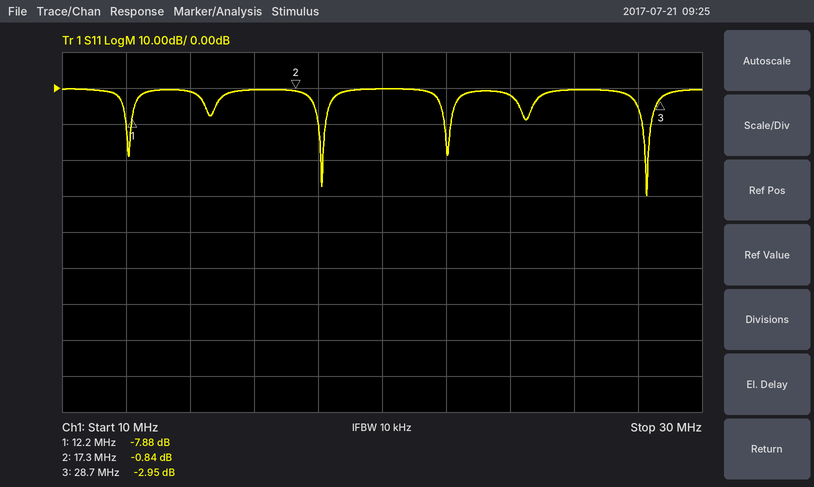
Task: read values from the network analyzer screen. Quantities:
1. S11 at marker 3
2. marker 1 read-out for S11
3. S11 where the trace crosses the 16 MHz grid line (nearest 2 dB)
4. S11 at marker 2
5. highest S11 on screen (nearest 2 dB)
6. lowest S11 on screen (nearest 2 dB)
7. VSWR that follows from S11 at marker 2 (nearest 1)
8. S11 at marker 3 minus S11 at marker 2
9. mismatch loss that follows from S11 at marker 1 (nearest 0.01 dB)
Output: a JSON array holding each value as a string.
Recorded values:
["-2.95 dB", "-7.88 dB", "0 dB", "-0.84 dB", "0 dB", "-30 dB", "21", "-2.11 dB", "0.77 dB"]
